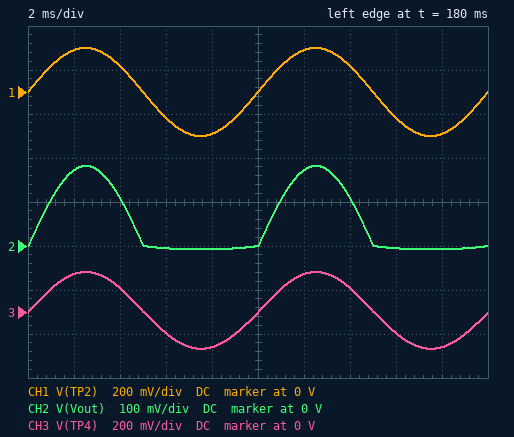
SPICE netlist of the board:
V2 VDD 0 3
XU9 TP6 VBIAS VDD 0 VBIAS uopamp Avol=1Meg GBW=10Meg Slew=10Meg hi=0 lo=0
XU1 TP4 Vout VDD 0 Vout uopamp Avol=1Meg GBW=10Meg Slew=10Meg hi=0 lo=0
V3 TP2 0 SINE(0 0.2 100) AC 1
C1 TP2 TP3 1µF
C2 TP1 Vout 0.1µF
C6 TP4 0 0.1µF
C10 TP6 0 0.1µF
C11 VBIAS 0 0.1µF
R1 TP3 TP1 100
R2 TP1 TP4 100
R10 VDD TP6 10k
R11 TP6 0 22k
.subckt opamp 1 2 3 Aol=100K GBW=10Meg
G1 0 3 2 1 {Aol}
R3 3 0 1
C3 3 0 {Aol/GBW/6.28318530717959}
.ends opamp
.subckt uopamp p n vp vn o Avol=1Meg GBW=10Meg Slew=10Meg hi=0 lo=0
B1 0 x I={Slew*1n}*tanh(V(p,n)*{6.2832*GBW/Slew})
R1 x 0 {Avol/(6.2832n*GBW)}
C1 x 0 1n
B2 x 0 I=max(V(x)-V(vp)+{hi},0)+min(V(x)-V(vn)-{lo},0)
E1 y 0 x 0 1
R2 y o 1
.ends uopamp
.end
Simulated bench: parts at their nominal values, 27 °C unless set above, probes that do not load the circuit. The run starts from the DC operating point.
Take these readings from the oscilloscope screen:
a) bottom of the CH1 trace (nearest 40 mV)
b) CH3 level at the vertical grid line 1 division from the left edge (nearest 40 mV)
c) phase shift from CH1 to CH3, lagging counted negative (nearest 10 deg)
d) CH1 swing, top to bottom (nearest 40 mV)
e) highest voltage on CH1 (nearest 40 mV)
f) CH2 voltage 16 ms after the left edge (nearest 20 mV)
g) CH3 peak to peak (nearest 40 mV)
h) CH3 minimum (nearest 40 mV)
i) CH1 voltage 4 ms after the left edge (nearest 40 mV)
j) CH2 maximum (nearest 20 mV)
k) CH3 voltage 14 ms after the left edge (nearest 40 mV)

-200 mV
160 mV
0 deg
400 mV
200 mV
0 V
360 mV
-160 mV
120 mV
180 mV
120 mV
